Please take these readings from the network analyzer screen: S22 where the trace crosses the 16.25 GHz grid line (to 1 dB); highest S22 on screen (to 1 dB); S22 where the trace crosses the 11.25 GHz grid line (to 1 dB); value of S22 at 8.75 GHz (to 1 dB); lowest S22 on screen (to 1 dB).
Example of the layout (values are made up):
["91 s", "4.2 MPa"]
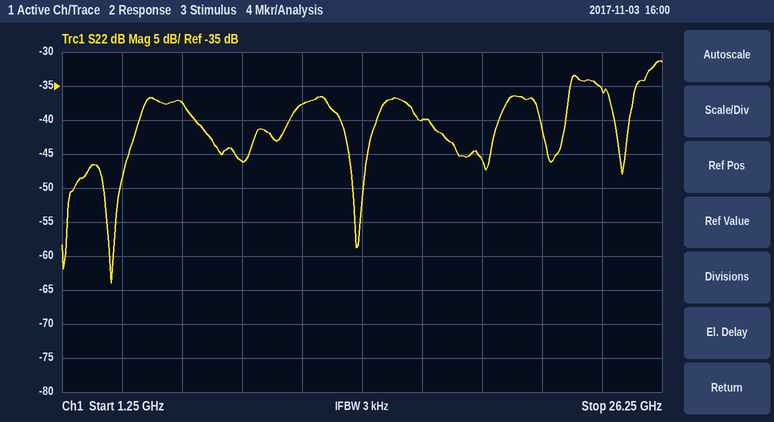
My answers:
["-40 dB", "-31 dB", "-38 dB", "-46 dB", "-64 dB"]
